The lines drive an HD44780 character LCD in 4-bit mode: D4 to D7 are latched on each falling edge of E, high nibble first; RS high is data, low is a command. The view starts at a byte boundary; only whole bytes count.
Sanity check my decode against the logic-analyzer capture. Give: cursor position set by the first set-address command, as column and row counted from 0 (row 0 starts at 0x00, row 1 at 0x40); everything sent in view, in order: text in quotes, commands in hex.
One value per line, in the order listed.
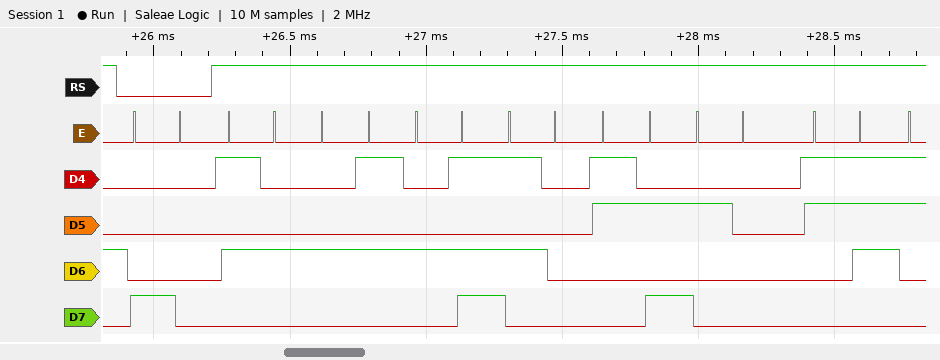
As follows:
column 0, row 0
0x80 "TEMP: 7"
